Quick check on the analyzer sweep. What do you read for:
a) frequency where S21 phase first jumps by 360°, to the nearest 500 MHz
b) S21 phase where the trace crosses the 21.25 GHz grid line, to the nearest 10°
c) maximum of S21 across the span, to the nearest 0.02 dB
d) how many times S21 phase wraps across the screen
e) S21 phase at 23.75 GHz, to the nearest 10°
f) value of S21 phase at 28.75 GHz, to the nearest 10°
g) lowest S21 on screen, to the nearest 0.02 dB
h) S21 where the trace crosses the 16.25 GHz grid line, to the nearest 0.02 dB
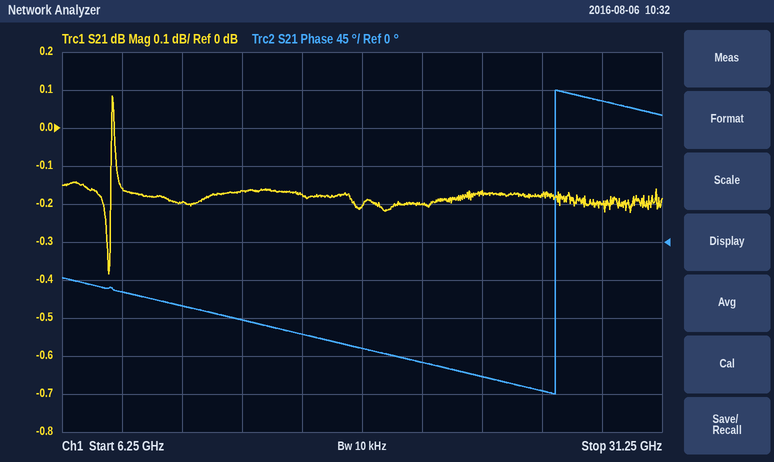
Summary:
27.0 GHz
-140°
0.08 dB
1
-160°
170°
-0.38 dB
-0.18 dB
